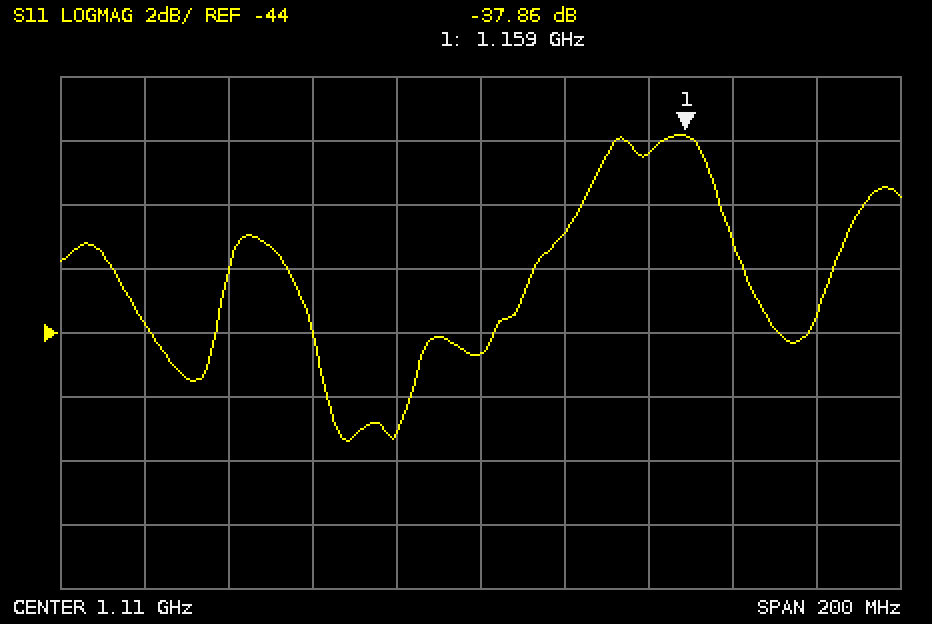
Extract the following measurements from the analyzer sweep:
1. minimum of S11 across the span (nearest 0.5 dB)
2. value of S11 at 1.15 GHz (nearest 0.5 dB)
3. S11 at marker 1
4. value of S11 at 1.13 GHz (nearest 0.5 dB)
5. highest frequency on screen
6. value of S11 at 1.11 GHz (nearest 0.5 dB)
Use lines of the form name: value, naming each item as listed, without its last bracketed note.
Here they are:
minimum of S11 across the span: -47.5 dB
value of S11 at 1.15 GHz: -38.5 dB
S11 at marker 1: -37.86 dB
value of S11 at 1.13 GHz: -41.0 dB
highest frequency on screen: 1.21 GHz
value of S11 at 1.11 GHz: -44.5 dB
